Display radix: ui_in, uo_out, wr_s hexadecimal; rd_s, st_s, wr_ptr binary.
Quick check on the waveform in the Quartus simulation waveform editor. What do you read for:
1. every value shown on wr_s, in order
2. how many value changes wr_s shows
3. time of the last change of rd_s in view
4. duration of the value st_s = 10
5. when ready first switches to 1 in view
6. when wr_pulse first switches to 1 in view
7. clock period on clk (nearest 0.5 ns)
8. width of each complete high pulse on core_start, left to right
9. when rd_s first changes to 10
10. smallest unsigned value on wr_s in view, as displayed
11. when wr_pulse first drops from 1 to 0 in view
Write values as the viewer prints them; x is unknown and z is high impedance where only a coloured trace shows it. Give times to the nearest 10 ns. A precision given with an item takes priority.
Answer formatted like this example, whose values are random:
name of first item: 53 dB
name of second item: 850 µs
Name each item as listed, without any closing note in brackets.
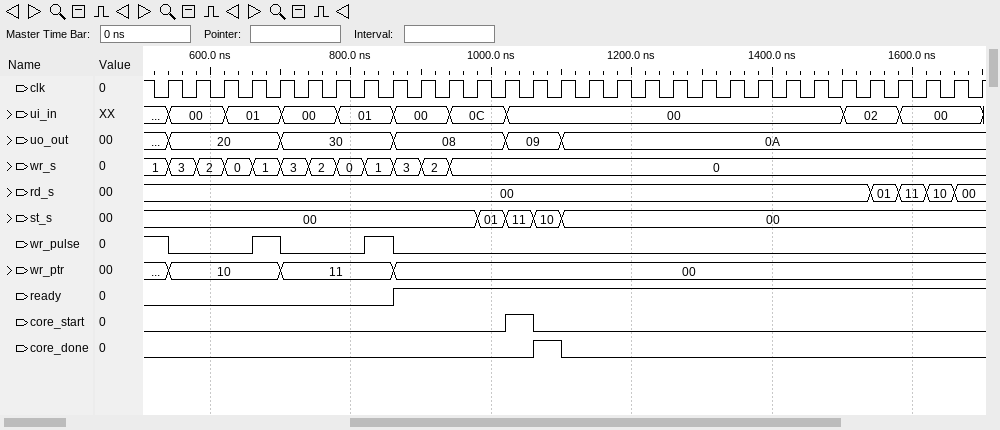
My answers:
every value shown on wr_s, in order: 1, 3, 2, 0, 1, 3, 2, 0, 1, 3, 2, 0
how many value changes wr_s shows: 11
time of the last change of rd_s in view: 1660 ns
duration of the value st_s = 10: 40 ns
when ready first switches to 1 in view: 860 ns
when wr_pulse first switches to 1 in view: 660 ns
clock period on clk: 40 ns
width of each complete high pulse on core_start, left to right: 40 ns
when rd_s first changes to 10: 1620 ns
smallest unsigned value on wr_s in view, as displayed: 0
when wr_pulse first drops from 1 to 0 in view: 540 ns
